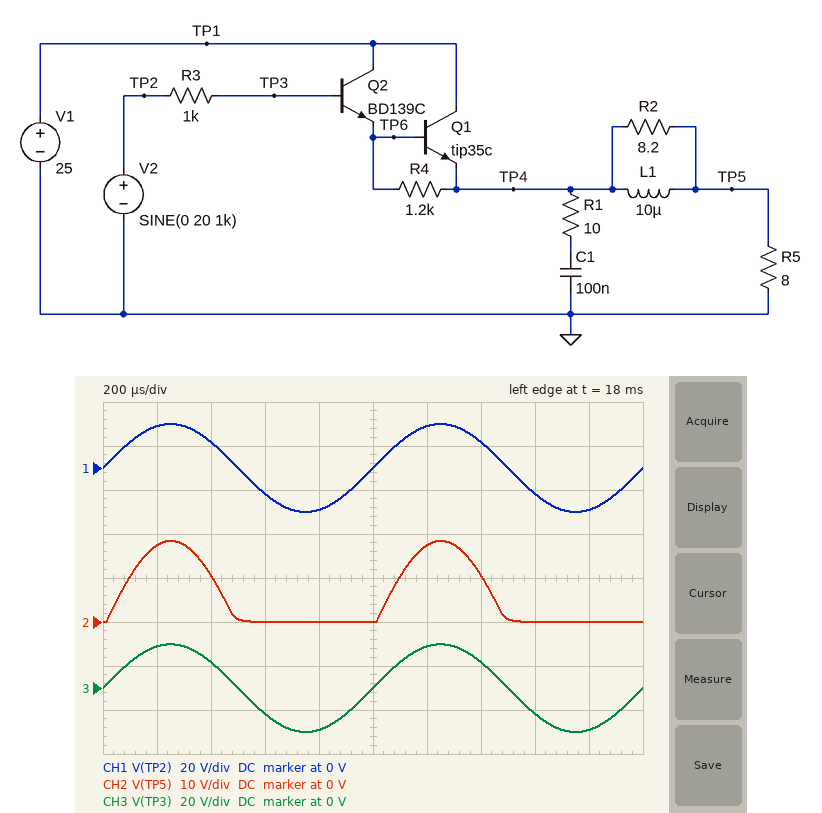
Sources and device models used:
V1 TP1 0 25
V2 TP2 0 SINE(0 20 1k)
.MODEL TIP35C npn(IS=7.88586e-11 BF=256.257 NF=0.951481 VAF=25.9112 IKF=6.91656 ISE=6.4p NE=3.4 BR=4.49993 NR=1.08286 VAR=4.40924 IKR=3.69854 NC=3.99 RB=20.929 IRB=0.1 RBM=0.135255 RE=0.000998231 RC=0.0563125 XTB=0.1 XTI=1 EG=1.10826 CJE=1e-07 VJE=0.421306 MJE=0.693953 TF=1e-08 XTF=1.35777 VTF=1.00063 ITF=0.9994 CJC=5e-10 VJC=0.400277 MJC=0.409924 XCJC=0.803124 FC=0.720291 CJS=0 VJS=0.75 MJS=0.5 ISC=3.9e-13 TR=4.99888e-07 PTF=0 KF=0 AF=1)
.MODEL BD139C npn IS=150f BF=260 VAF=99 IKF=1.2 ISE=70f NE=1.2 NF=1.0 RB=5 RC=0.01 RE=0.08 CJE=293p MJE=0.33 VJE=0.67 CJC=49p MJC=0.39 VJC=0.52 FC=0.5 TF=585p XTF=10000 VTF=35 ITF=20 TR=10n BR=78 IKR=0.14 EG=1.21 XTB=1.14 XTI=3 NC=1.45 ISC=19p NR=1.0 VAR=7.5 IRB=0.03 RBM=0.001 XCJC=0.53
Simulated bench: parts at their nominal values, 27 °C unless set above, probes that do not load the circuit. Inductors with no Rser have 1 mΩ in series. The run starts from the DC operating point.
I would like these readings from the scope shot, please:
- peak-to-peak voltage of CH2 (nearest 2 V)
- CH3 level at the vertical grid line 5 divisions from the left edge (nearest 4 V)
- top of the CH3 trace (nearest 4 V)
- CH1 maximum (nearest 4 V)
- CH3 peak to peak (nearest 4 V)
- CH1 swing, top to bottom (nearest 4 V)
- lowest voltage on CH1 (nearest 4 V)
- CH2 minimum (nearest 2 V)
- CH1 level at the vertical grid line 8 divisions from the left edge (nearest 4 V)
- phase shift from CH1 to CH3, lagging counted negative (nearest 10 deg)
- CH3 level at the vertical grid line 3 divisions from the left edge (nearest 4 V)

18 V
0 V
20 V
20 V
40 V
40 V
-20 V
0 V
-12 V
0 deg
-12 V
